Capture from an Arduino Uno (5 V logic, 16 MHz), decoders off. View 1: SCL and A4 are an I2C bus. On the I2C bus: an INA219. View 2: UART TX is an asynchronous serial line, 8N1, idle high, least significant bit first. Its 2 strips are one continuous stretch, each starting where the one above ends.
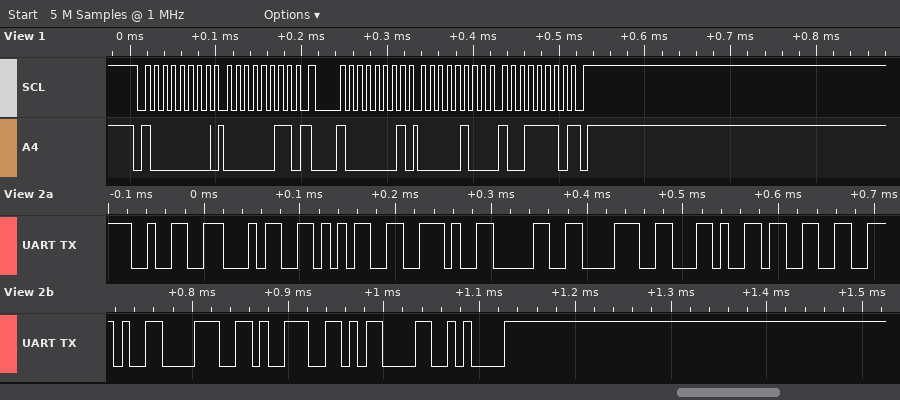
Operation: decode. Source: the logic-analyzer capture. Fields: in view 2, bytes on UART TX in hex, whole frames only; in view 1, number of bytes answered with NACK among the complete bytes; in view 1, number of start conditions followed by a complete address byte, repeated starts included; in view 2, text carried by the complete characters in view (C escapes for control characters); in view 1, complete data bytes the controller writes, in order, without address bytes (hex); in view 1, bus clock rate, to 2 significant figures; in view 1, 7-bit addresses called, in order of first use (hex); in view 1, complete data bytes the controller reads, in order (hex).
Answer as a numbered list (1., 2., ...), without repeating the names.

1. 32 34 35 2E 30 38 2C 33 2E 38 39 0D 0A
2. 1
3. 2
4. "245.08,3.89\r\n"
5. 03
6. 100 kHz
7. 0x40
8. 04 9E
